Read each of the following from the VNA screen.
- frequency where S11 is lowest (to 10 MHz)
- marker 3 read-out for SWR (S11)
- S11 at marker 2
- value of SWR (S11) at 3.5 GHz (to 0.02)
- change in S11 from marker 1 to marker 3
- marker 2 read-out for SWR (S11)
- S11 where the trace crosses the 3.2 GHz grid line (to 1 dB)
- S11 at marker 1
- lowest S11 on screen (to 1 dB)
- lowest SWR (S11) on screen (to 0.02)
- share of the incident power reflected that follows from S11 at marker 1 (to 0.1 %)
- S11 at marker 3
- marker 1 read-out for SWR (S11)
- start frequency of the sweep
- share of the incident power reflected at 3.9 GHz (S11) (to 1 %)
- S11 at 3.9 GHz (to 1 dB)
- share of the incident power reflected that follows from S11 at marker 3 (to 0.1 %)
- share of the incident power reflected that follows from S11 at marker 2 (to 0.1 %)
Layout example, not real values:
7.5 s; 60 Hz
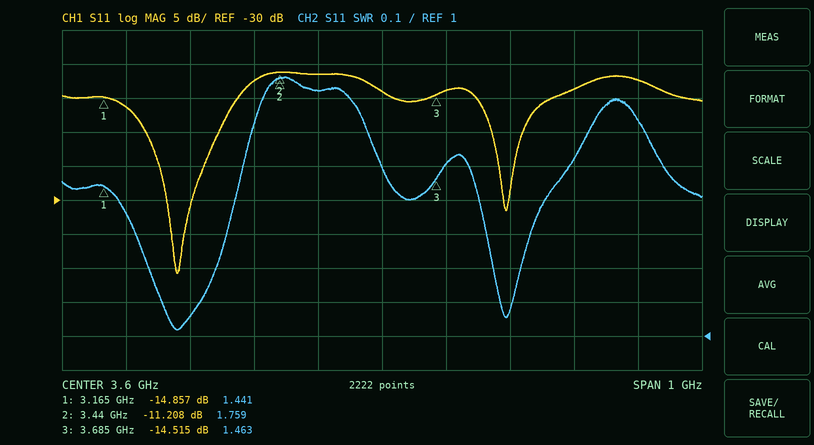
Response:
3.28 GHz; 1.463; -11.208 dB; 1.72; 0.342 dB; 1.759; -16 dB; -14.857 dB; -41 dB; 1.02; 3.3 %; -14.515 dB; 1.441; 3.1 GHz; 4 %; -14 dB; 3.5 %; 7.6 %
